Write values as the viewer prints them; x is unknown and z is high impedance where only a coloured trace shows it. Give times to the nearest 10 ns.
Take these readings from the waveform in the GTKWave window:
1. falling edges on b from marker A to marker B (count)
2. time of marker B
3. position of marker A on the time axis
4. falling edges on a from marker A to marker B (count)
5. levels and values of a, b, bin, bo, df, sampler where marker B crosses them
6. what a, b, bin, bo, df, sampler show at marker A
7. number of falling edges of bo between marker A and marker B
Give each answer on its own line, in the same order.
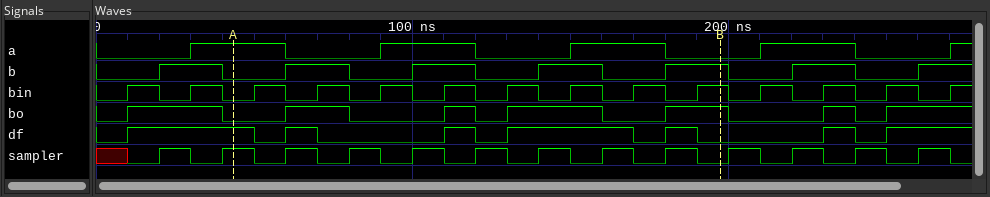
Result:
3
200 ns
40 ns
3
a=0, b=1, bin=1, bo=1, df=0, sampler=0
a=1, b=0, bin=0, bo=0, df=1, sampler=1
3
